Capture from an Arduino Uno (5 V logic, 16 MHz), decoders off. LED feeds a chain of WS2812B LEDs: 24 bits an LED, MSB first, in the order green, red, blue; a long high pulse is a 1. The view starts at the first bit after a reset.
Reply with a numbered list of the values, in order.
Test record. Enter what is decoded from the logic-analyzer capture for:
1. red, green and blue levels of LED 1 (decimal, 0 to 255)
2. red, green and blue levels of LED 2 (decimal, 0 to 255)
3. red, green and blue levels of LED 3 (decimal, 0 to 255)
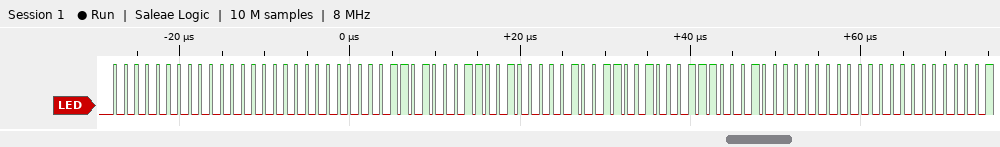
1. 0, 0, 0
2. 100, 52, 19
3. 136, 35, 0
